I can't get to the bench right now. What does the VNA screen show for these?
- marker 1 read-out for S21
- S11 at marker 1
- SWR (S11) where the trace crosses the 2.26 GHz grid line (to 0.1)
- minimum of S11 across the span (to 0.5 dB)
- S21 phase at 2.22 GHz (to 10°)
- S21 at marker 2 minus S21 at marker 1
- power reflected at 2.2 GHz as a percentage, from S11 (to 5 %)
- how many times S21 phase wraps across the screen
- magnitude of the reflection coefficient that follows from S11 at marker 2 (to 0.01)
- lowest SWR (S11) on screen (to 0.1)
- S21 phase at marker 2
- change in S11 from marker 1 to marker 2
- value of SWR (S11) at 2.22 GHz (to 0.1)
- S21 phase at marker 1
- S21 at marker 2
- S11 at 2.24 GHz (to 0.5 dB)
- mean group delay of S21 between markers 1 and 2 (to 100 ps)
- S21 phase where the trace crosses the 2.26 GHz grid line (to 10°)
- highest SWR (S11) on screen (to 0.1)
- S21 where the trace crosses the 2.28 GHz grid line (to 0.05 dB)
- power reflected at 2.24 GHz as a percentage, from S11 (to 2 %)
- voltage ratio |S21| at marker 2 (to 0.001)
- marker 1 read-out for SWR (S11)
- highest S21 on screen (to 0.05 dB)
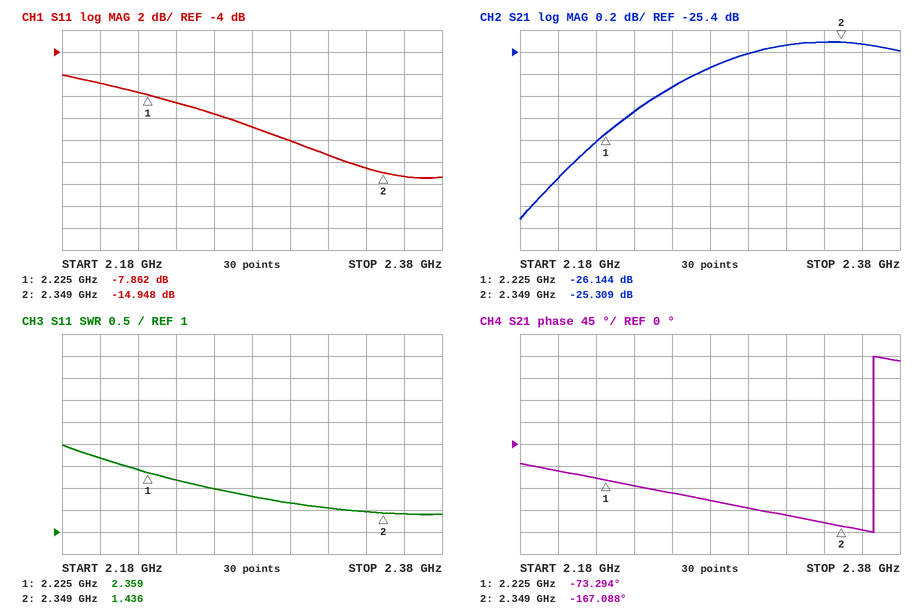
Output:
-26.144 dB
-7.862 dB
2.0
-15.5 dB
-70°
0.835 dB
20 %
1
0.18
1.4
-167.088°
-7.086 dB
2.4
-73.294°
-25.309 dB
-8.5 dB
2.1 ns
-100°
3.0
-25.55 dB
14 %
0.054
2.359
-25.30 dB
